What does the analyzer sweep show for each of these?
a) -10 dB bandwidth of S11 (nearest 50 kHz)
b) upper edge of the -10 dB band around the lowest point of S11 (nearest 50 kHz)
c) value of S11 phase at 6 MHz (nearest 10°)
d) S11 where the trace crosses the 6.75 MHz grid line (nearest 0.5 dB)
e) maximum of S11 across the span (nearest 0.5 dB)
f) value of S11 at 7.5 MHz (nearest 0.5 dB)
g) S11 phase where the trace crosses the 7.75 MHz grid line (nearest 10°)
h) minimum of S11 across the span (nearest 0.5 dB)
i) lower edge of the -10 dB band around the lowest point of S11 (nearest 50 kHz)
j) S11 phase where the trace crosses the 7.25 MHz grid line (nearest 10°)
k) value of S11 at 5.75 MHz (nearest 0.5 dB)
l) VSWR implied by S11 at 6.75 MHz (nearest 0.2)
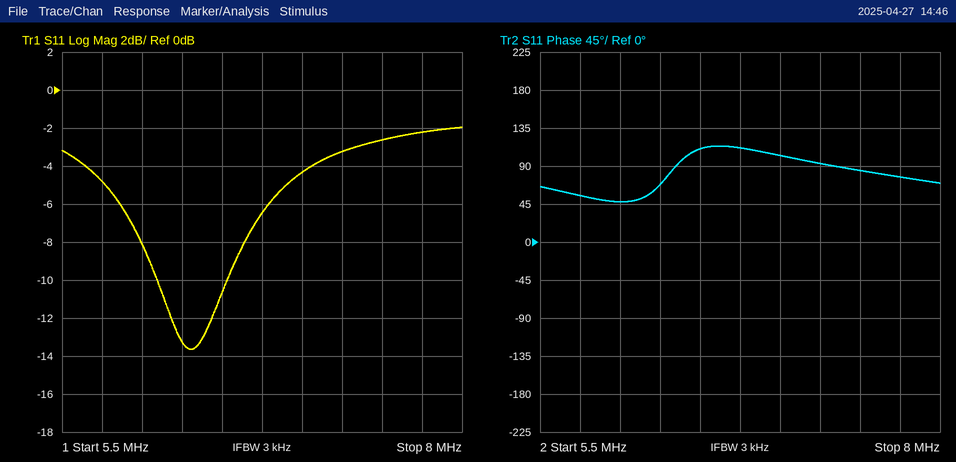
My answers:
450 kHz
6.55 MHz
50°
-6.5 dB
-2.0 dB
-2.5 dB
80°
-13.5 dB
6.10 MHz
90°
-5.0 dB
2.8
